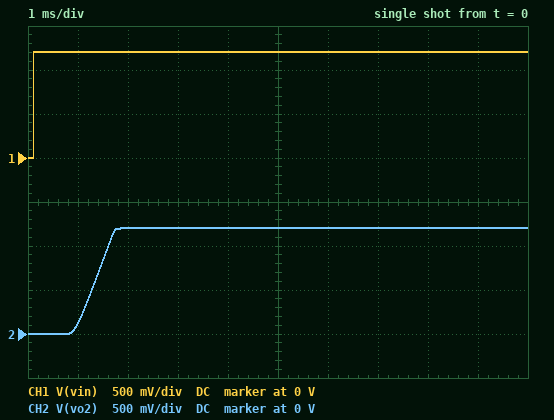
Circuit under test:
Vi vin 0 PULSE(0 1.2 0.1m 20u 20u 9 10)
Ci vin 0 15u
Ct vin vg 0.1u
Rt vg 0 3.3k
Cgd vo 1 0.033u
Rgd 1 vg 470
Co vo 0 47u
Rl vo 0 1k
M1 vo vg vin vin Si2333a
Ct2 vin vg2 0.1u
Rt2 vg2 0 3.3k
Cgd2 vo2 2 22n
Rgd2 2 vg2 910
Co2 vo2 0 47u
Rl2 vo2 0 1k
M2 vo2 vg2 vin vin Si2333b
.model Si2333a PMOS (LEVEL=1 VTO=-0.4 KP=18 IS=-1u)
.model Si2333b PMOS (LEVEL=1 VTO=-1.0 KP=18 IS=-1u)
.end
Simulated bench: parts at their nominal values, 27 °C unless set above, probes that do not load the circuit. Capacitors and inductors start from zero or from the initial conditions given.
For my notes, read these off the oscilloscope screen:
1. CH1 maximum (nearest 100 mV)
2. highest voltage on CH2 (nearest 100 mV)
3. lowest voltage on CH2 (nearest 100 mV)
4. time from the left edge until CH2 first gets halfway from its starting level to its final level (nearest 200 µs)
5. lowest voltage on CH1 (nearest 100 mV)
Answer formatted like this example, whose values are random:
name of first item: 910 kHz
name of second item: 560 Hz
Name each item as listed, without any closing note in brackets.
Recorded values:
CH1 maximum: 1.2 V
highest voltage on CH2: 1.2 V
lowest voltage on CH2: 0 V
time from the left edge until CH2 first gets halfway from its starting level to its final level: 1.4 ms
lowest voltage on CH1: 0 V
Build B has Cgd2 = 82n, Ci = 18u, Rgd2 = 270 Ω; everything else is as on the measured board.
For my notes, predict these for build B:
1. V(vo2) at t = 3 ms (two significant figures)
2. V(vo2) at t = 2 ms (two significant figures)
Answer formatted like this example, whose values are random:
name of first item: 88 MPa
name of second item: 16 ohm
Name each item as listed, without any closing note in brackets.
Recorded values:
V(vo2) at t = 3 ms: 1.1 V
V(vo2) at t = 2 ms: 550 mV
